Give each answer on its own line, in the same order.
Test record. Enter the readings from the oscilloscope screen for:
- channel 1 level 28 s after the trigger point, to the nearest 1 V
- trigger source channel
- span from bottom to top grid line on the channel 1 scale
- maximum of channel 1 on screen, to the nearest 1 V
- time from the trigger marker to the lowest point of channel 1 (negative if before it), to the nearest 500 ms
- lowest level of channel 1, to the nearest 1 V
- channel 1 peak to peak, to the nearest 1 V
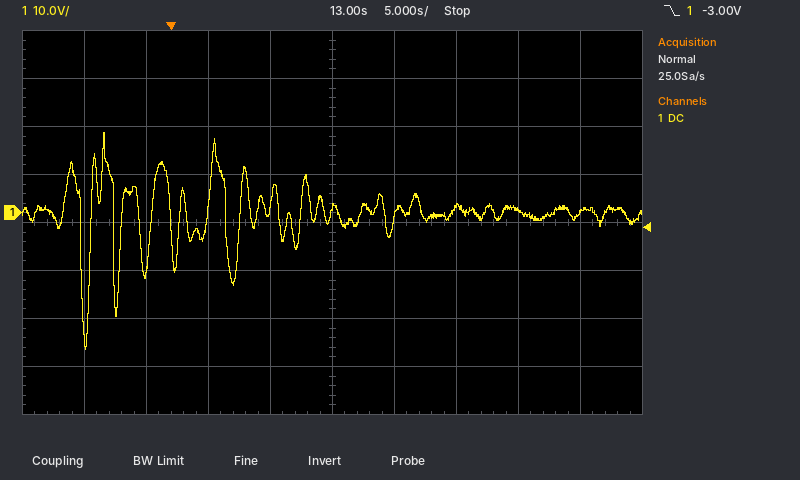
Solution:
1 V
channel 1
80 V
17 V
-7.0 s
-28 V
45 V
